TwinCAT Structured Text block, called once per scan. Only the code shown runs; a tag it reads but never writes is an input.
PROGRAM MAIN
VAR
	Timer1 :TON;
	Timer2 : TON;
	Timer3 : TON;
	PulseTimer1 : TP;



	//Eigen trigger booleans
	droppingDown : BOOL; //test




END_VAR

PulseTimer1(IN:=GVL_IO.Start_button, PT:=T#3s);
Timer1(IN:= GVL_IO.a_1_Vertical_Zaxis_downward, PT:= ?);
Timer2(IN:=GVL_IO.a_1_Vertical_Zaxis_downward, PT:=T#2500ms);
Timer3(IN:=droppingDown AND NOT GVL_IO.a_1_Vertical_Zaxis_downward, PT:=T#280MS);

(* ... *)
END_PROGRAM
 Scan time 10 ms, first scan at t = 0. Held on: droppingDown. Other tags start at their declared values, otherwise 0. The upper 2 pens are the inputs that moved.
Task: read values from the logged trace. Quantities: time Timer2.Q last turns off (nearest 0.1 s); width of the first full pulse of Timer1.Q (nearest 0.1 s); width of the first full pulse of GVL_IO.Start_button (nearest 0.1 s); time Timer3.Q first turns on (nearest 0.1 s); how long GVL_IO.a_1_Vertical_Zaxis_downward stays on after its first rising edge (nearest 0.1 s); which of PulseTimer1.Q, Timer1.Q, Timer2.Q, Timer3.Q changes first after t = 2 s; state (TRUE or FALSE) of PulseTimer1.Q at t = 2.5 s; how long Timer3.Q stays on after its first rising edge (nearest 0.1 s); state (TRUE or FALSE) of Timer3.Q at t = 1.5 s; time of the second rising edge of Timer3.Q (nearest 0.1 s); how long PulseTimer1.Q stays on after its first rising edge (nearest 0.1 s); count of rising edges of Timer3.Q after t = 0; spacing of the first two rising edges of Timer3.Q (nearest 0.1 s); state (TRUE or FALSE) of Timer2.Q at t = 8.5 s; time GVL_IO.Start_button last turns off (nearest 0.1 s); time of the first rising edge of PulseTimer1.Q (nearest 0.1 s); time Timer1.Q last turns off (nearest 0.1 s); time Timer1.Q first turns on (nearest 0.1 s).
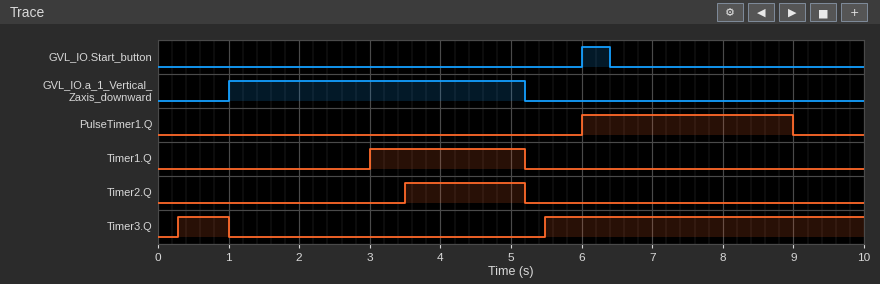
5.2 s
2.2 s
0.4 s
0.3 s
4.2 s
Timer1.Q
FALSE
0.7 s
FALSE
5.5 s
3.0 s
2
5.2 s
FALSE
6.4 s
6.0 s
5.2 s
3.0 s
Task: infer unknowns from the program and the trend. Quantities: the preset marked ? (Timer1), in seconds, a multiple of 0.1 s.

2.0 s
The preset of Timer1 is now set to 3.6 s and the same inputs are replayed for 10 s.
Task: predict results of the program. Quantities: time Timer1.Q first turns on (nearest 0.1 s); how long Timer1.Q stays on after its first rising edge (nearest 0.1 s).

4.6 s
0.6 s
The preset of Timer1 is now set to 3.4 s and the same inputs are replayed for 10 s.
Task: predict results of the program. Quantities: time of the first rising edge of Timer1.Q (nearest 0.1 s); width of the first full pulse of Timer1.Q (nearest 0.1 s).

4.4 s
0.8 s
